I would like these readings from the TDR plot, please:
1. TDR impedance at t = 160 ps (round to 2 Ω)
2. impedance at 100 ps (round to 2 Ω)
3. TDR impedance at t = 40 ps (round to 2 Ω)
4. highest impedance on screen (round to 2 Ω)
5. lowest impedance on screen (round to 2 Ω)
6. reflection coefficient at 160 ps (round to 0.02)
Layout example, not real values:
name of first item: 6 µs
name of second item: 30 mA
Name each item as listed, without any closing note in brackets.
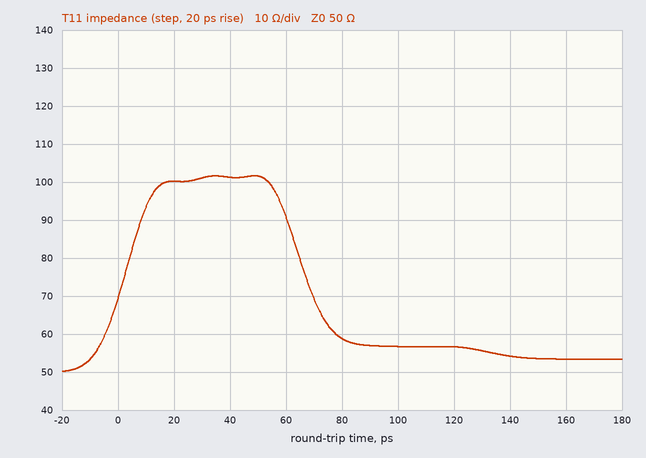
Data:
TDR impedance at t = 160 ps: 54 Ω
impedance at 100 ps: 56 Ω
TDR impedance at t = 40 ps: 102 Ω
highest impedance on screen: 102 Ω
lowest impedance on screen: 50 Ω
reflection coefficient at 160 ps: +0.04
